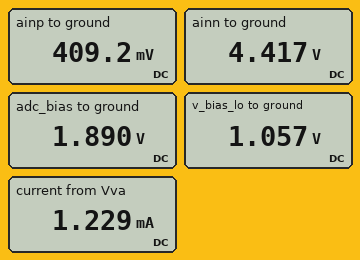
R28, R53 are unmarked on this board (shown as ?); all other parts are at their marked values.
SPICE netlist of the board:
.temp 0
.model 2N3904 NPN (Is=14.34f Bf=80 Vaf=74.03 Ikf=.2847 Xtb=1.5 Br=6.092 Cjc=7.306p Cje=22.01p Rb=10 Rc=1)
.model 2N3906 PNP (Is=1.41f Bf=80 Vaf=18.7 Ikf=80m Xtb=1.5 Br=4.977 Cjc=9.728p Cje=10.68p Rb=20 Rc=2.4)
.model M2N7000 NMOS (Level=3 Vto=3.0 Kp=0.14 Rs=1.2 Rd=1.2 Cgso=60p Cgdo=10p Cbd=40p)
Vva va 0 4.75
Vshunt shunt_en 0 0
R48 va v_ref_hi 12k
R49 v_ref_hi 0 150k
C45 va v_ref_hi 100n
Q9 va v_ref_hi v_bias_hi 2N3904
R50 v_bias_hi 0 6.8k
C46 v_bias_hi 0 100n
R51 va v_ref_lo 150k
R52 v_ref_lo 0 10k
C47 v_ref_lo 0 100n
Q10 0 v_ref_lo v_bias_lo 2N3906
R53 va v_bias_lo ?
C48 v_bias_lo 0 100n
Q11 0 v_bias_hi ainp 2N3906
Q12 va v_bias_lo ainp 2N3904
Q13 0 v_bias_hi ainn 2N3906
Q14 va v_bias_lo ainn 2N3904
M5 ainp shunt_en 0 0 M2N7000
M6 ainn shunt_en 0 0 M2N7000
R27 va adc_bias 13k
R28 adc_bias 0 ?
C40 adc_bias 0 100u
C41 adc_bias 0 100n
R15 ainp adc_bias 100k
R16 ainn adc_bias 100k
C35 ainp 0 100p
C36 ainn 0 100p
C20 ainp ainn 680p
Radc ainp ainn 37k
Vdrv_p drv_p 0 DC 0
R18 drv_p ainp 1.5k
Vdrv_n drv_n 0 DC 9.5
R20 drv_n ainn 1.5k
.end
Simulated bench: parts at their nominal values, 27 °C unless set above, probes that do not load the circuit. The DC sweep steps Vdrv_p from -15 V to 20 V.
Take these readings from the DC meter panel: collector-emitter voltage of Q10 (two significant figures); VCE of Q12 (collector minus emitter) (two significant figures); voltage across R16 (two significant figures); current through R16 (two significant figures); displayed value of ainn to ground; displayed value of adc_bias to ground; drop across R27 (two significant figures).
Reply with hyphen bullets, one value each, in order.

- -1.1 V
- 4.3 V
- 2.5 V
- 25 µA
- 4.417 V
- 1.890 V
- 2.9 V
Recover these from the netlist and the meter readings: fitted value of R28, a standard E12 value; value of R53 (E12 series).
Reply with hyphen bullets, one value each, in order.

- 8.2 kΩ
- 12 kΩ
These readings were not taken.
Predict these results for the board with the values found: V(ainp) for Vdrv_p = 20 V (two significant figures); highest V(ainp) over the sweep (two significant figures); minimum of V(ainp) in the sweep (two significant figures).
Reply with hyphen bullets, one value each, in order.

- 4.5 V
- 4.5 V
- 280 mV
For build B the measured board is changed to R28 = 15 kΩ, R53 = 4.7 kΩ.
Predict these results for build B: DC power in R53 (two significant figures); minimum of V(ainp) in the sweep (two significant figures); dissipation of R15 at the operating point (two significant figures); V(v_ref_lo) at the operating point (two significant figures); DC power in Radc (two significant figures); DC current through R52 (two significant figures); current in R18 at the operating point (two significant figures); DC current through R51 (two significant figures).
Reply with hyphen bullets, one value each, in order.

- 2.8 mW
- 370 mV
- 42 µW
- 400 mV
- 420 µW
- 40 µA
- 320 µA
- 29 µA
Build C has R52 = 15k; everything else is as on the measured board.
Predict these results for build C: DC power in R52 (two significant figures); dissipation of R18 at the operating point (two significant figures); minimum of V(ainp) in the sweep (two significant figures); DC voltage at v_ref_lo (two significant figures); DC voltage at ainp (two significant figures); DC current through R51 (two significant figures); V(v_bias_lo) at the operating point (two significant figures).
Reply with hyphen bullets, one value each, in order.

- 16 µW
- 200 µW
- 420 mV
- 490 mV
- 550 mV
- 28 µA
- 1.2 V
